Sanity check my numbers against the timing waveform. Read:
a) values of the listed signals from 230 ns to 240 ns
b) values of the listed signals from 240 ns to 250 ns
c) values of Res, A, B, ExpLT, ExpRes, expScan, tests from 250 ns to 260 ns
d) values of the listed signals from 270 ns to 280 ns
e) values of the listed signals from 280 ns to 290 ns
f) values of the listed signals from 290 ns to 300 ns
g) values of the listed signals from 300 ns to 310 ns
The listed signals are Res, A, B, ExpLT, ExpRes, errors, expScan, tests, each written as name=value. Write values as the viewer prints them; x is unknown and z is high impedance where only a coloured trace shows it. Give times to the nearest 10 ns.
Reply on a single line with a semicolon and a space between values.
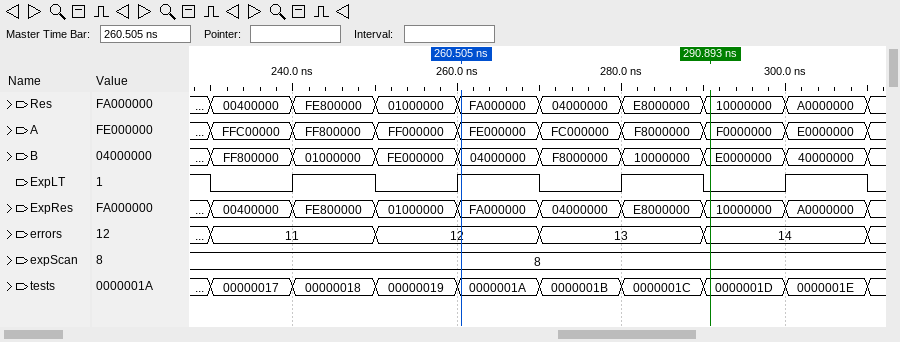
Res=00400000, A=FFC00000, B=FF800000, ExpLT=0, ExpRes=00400000, errors=11, expScan=8, tests=00000017; Res=FE800000, A=FF800000, B=01000000, ExpLT=1, ExpRes=FE800000, errors=11, expScan=8, tests=00000018; Res=01000000, A=FF000000, B=FE000000, ExpLT=0, ExpRes=01000000, expScan=8, tests=00000019; Res=04000000, A=FC000000, B=F8000000, ExpLT=0, ExpRes=04000000, errors=13, expScan=8, tests=0000001B; Res=E8000000, A=F8000000, B=10000000, ExpLT=1, ExpRes=E8000000, errors=13, expScan=8, tests=0000001C; Res=10000000, A=F0000000, B=E0000000, ExpLT=0, ExpRes=10000000, errors=14, expScan=8, tests=0000001D; Res=A0000000, A=E0000000, B=40000000, ExpLT=1, ExpRes=A0000000, errors=14, expScan=8, tests=0000001E
